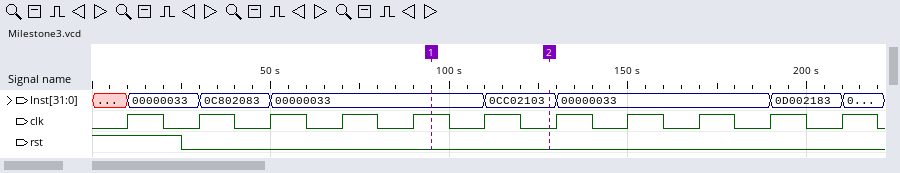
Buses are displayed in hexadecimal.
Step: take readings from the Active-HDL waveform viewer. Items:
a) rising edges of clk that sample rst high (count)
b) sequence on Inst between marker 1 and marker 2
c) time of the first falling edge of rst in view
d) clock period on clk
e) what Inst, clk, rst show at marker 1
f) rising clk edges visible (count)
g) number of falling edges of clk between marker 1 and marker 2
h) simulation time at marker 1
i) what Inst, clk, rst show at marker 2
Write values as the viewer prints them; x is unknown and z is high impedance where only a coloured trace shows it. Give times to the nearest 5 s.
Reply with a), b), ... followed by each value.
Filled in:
a) 1
b) 00000033, 0CC02103
c) 25 s
d) 20 s
e) Inst=00000033, clk=1, rst=0
f) 11
g) 2
h) 95 s
i) Inst=0CC02103, clk=0, rst=0
